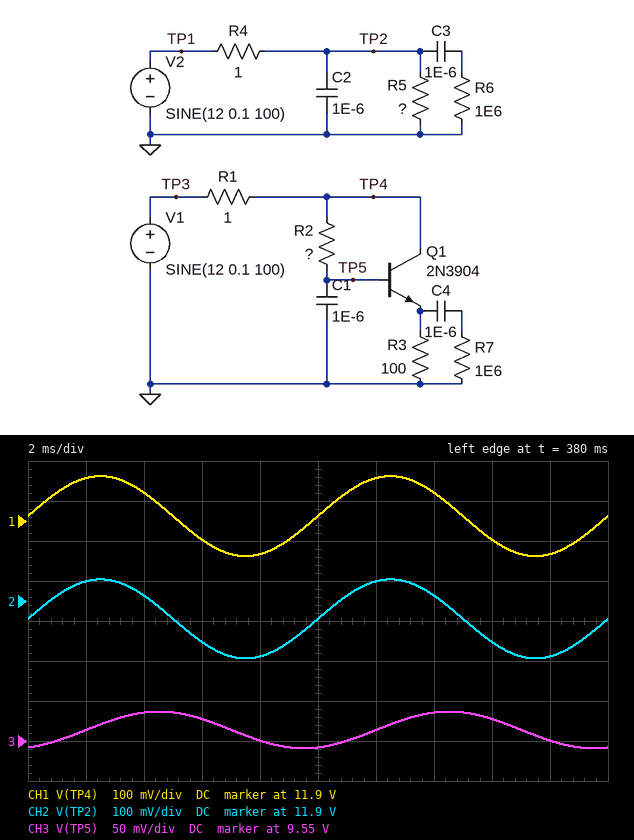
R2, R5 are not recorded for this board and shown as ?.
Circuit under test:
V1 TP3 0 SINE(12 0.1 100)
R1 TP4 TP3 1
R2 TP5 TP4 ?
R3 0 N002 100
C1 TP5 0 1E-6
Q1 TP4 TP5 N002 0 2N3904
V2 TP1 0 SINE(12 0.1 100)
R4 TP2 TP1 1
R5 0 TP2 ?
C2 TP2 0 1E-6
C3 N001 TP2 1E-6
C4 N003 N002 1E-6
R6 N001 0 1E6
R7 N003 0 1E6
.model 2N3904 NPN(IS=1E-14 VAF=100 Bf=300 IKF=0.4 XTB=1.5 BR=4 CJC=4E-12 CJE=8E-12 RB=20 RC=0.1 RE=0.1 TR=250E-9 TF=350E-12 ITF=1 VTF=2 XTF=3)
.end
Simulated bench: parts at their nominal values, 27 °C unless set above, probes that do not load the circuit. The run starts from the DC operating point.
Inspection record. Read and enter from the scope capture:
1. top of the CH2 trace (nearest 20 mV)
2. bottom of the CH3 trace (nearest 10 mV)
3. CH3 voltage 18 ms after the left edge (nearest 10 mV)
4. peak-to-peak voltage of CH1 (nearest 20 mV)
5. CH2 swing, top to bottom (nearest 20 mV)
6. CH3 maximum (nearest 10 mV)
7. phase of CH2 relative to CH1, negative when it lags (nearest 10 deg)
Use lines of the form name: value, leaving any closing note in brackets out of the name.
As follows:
top of the CH2 trace: 11.96 V
bottom of the CH3 trace: 9.54 V
CH3 voltage 18 ms after the left edge: 9.55 V
peak-to-peak voltage of CH1: 200 mV
CH2 swing, top to bottom: 200 mV
CH3 maximum: 9.59 V
phase of CH2 relative to CH1, negative when it lags: 0 deg
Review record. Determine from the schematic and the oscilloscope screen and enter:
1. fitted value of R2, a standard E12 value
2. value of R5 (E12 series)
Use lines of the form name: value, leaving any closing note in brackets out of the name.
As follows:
fitted value of R2, a standard E12 value: 6.8 kΩ
value of R5: 82 Ω
